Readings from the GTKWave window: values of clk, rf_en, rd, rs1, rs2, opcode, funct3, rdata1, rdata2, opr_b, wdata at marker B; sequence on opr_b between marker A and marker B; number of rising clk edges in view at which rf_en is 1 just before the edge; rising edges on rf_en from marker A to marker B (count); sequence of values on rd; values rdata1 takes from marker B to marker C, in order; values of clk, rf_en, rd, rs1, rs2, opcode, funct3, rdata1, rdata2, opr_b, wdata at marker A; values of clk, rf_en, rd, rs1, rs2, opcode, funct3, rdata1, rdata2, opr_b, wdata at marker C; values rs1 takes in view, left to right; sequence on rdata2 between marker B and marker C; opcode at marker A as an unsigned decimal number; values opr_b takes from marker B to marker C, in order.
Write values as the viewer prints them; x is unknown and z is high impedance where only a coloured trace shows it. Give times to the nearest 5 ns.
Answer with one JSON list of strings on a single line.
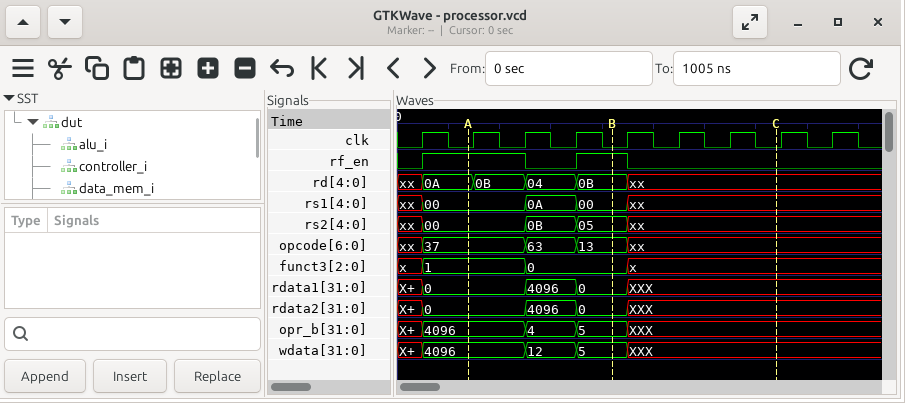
["clk=0, rf_en=1, rd=0B, rs1=00, rs2=05, opcode=13, funct3=0, rdata1=0, rdata2=0, opr_b=5, wdata=5", "4096, 4, 5", "3", "1", "xx, 0A, 0B, 04, 0B, xx", "0, XXX", "clk=0, rf_en=1, rd=0A, rs1=00, rs2=00, opcode=37, funct3=1, rdata1=0, rdata2=0, opr_b=4096, wdata=4096", "clk=0, rf_en=0, rd=xx, rs1=xx, rs2=xx, opcode=xx, funct3=x, rdata1=XXX, rdata2=XXX, opr_b=XXX, wdata=XXX", "xx, 00, 0A, 00, xx", "0, XXX", "55", "5, XXX"]
